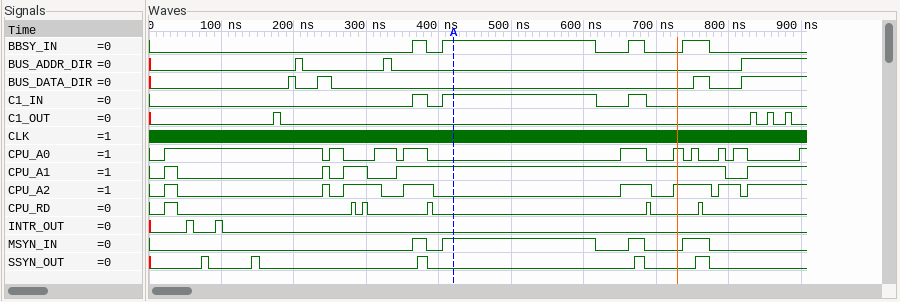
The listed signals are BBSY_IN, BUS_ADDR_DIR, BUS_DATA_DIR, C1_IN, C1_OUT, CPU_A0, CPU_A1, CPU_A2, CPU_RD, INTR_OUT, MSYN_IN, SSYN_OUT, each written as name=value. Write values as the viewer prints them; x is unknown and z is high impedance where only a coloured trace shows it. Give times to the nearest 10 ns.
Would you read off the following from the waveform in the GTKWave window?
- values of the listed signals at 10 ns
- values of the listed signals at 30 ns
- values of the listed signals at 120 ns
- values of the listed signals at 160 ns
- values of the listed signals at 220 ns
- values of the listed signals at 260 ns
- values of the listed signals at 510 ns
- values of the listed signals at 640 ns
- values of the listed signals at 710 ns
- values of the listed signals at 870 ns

BBSY_IN=0, BUS_ADDR_DIR=0, BUS_DATA_DIR=0, C1_IN=0, C1_OUT=0, CPU_A0=0, CPU_A1=0, CPU_A2=0, CPU_RD=0, INTR_OUT=0, MSYN_IN=0, SSYN_OUT=0
BBSY_IN=0, BUS_ADDR_DIR=0, BUS_DATA_DIR=0, C1_IN=0, C1_OUT=0, CPU_A0=1, CPU_A1=1, CPU_A2=1, CPU_RD=1, INTR_OUT=0, MSYN_IN=0, SSYN_OUT=0
BBSY_IN=0, BUS_ADDR_DIR=0, BUS_DATA_DIR=0, C1_IN=0, C1_OUT=0, CPU_A0=1, CPU_A1=0, CPU_A2=0, CPU_RD=0, INTR_OUT=0, MSYN_IN=0, SSYN_OUT=0
BBSY_IN=0, BUS_ADDR_DIR=0, BUS_DATA_DIR=0, C1_IN=0, C1_OUT=0, CPU_A0=1, CPU_A1=0, CPU_A2=0, CPU_RD=0, INTR_OUT=0, MSYN_IN=0, SSYN_OUT=0
BBSY_IN=0, BUS_ADDR_DIR=0, BUS_DATA_DIR=0, C1_IN=0, C1_OUT=0, CPU_A0=1, CPU_A1=0, CPU_A2=0, CPU_RD=0, INTR_OUT=0, MSYN_IN=0, SSYN_OUT=0
BBSY_IN=0, BUS_ADDR_DIR=0, BUS_DATA_DIR=0, C1_IN=0, C1_OUT=0, CPU_A0=1, CPU_A1=0, CPU_A2=0, CPU_RD=0, INTR_OUT=0, MSYN_IN=0, SSYN_OUT=0
BBSY_IN=1, BUS_ADDR_DIR=0, BUS_DATA_DIR=0, C1_IN=1, C1_OUT=0, CPU_A0=0, CPU_A1=1, CPU_A2=0, CPU_RD=0, INTR_OUT=0, MSYN_IN=1, SSYN_OUT=0
BBSY_IN=0, BUS_ADDR_DIR=0, BUS_DATA_DIR=0, C1_IN=0, C1_OUT=0, CPU_A0=0, CPU_A1=1, CPU_A2=0, CPU_RD=0, INTR_OUT=0, MSYN_IN=0, SSYN_OUT=0
BBSY_IN=0, BUS_ADDR_DIR=0, BUS_DATA_DIR=0, C1_IN=0, C1_OUT=0, CPU_A0=0, CPU_A1=1, CPU_A2=0, CPU_RD=0, INTR_OUT=0, MSYN_IN=0, SSYN_OUT=0
BBSY_IN=0, BUS_ADDR_DIR=1, BUS_DATA_DIR=1, C1_IN=0, C1_OUT=0, CPU_A0=0, CPU_A1=1, CPU_A2=1, CPU_RD=0, INTR_OUT=0, MSYN_IN=0, SSYN_OUT=0
